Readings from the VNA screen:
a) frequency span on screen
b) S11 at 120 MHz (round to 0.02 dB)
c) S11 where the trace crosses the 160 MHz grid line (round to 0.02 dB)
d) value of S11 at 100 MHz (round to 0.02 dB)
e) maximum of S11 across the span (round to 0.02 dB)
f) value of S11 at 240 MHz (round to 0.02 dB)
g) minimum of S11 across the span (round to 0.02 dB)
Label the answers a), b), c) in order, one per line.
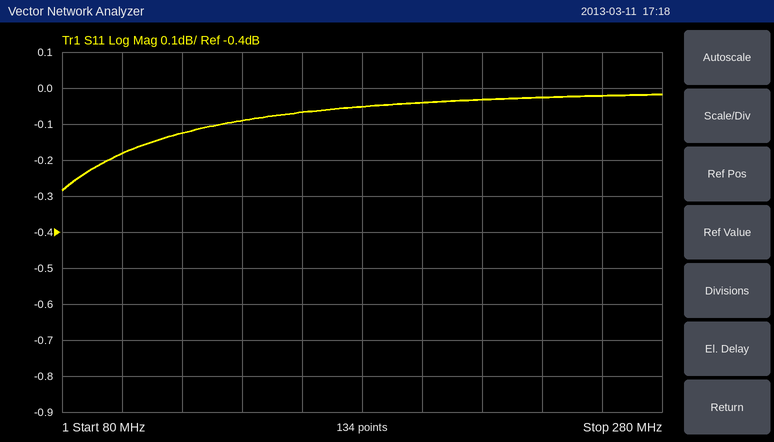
a) 200 MHz
b) -0.12 dB
c) -0.06 dB
d) -0.18 dB
e) -0.02 dB
f) -0.02 dB
g) -0.28 dB
